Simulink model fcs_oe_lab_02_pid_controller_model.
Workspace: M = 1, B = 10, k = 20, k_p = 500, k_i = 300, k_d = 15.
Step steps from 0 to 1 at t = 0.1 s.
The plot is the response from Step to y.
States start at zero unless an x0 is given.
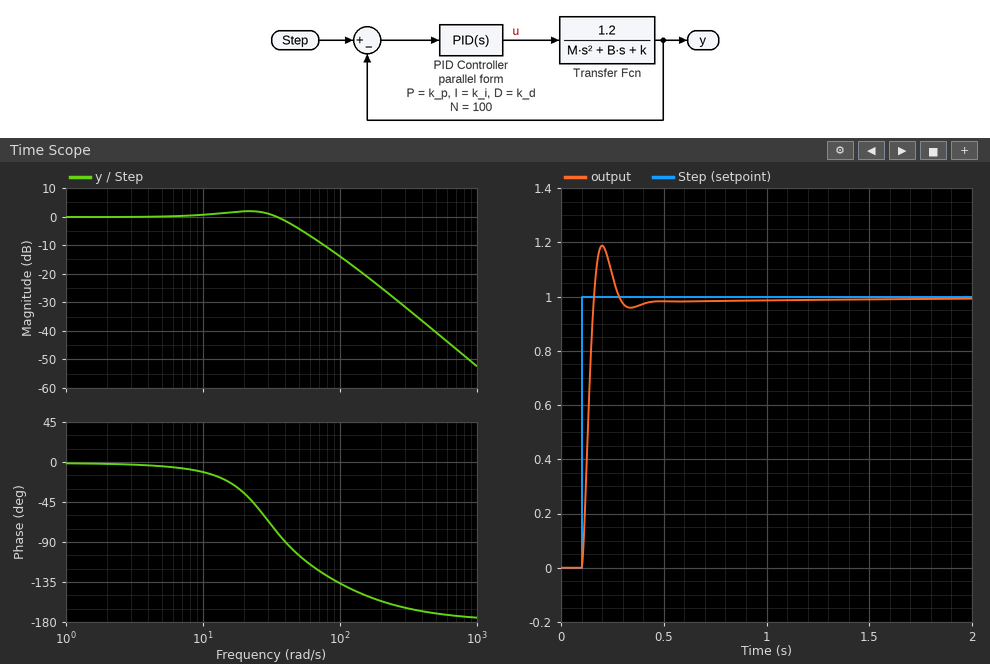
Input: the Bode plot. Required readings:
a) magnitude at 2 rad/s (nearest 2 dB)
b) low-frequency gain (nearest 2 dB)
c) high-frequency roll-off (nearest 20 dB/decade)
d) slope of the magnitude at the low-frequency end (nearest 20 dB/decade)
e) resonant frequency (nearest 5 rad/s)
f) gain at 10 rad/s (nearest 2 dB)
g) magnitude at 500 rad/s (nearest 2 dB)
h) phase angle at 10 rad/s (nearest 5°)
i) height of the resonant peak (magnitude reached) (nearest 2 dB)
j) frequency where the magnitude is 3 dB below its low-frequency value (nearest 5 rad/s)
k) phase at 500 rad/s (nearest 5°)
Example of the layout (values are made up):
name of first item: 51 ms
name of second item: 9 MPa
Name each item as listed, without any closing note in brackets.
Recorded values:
magnitude at 2 rad/s: 0 dB
low-frequency gain: 0 dB
high-frequency roll-off: -40 dB/decade
slope of the magnitude at the low-frequency end: 0 dB/decade
resonant frequency: 20 rad/s
gain at 10 rad/s: 0 dB
magnitude at 500 rad/s: -40 dB
phase angle at 10 rad/s: -10°
height of the resonant peak (magnitude reached): 2 dB
frequency where the magnitude is 3 dB below its low-frequency value: 45 rad/s
phase at 500 rad/s: -170°
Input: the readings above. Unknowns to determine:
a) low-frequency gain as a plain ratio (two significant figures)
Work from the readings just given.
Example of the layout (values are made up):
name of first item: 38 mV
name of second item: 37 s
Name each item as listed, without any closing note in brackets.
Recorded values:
low-frequency gain as a plain ratio: 1.0
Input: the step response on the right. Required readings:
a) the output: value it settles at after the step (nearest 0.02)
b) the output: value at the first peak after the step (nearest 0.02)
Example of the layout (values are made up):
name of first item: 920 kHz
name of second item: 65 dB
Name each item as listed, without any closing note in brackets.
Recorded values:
the output: value it settles at after the step: 1.00
the output: value at the first peak after the step: 1.18
